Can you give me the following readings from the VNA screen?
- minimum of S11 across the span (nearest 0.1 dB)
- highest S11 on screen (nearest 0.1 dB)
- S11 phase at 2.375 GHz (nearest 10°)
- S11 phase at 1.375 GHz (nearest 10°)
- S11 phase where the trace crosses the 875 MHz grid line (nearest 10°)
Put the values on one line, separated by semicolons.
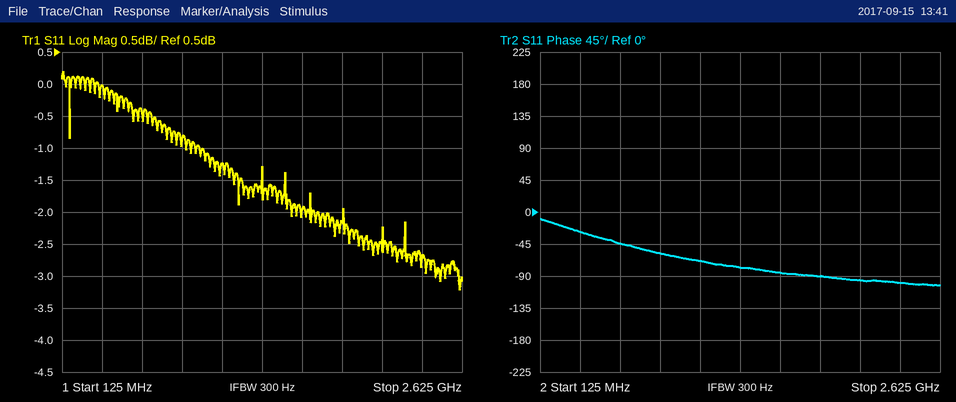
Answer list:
-3.2 dB; 0.2 dB; -100°; -80°; -60°
